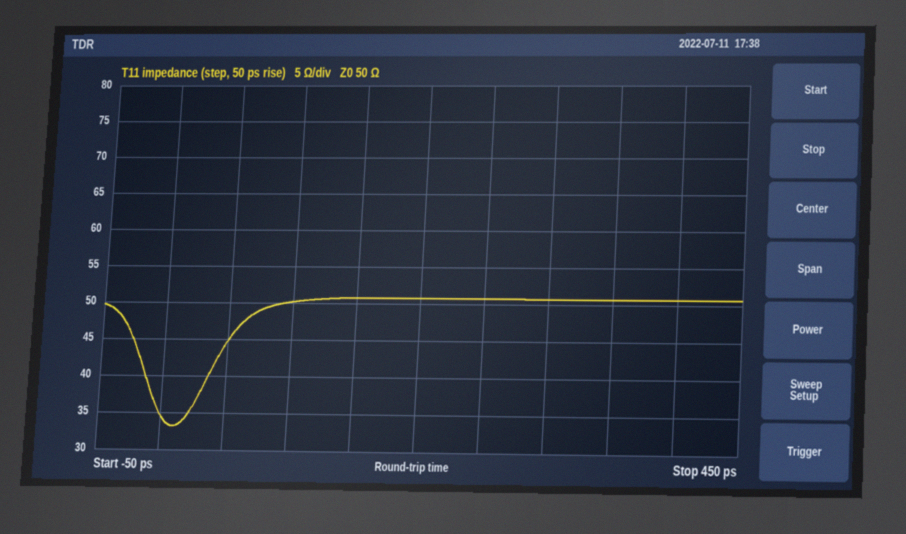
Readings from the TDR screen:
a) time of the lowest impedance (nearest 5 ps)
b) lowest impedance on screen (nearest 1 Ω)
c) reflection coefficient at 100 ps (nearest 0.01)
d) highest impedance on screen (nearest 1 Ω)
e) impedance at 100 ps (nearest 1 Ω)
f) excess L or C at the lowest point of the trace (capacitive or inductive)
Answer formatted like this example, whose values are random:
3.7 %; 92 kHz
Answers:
10 ps; 33 Ω; 0.00; 51 Ω; 50 Ω; capacitive
